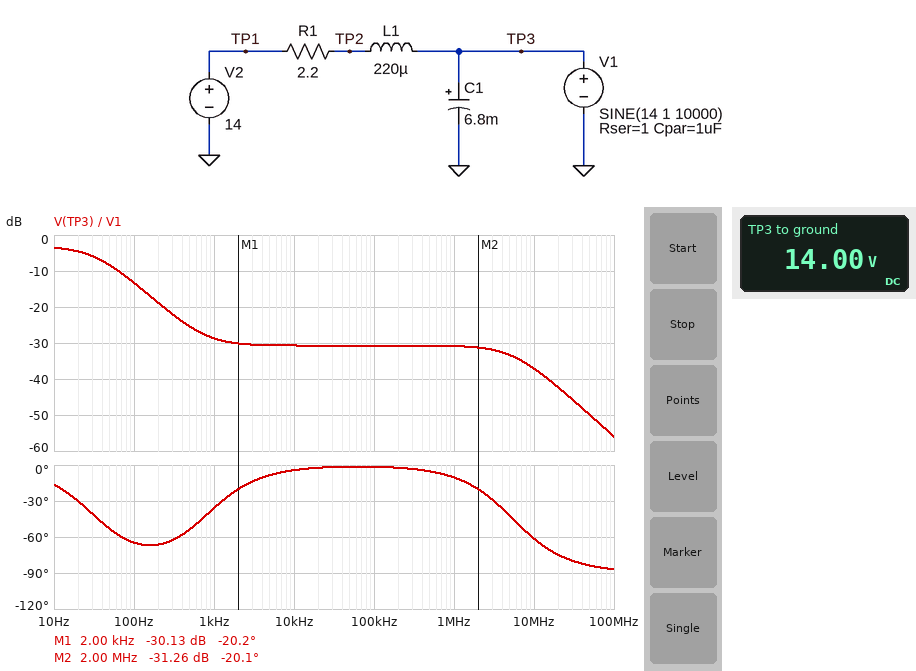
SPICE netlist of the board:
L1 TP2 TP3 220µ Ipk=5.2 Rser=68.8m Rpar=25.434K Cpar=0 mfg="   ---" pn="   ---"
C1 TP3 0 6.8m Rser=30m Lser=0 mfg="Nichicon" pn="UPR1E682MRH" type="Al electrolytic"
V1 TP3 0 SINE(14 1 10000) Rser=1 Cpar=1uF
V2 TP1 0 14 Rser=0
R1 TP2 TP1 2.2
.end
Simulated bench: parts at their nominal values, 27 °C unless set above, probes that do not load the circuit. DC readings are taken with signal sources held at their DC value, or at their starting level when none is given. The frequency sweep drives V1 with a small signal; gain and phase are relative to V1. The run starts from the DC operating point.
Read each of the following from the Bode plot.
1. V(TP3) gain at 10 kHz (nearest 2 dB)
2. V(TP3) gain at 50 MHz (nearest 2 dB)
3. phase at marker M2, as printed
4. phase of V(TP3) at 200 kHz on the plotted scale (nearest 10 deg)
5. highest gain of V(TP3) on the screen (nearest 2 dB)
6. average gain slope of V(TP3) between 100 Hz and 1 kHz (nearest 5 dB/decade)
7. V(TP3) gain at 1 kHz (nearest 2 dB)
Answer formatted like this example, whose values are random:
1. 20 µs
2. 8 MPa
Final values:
1. -30 dB
2. -50 dB
3. -20.1 deg
4. 0 deg
5. -4 dB
6. -15 dB/decade
7. -28 dB
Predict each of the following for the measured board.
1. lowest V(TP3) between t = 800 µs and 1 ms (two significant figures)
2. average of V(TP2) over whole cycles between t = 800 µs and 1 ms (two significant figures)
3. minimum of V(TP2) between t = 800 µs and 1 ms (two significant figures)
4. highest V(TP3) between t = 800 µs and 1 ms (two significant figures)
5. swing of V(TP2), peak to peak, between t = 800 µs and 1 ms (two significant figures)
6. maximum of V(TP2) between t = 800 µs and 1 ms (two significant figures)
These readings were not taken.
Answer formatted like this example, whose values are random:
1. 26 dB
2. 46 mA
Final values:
1. 14 V
2. 14 V
3. 14 V
4. 14 V
5. 9.2 mV
6. 14 V
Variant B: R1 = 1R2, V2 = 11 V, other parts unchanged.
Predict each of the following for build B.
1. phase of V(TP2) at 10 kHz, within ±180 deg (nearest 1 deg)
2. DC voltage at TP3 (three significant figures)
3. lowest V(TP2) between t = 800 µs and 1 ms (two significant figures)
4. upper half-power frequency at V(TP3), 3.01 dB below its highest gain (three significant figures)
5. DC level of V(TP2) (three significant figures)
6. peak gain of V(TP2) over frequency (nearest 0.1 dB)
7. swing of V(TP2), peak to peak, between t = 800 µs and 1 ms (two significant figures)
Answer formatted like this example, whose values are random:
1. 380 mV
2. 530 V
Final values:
1. -89 deg
2. 12.7 V
3. 13 V
4. 40.6 Hz
5. 12.6 V
6. -5.5 dB
7. 5.1 mV
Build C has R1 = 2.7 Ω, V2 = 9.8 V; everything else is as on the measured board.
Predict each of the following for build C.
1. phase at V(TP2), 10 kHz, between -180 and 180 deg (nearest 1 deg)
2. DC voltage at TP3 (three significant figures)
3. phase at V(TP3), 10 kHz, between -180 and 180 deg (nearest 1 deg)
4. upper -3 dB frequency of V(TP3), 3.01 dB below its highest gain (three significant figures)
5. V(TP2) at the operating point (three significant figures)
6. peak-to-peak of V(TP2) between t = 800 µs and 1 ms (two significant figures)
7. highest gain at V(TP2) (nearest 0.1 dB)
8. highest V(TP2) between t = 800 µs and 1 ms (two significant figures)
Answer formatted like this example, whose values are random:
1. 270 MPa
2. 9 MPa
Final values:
1. -83 deg
2. 12.9 V
3. -4 deg
4. 30.8 Hz
5. 12.8 V
6. 11 mV
7. -2.9 dB
8. 13 V
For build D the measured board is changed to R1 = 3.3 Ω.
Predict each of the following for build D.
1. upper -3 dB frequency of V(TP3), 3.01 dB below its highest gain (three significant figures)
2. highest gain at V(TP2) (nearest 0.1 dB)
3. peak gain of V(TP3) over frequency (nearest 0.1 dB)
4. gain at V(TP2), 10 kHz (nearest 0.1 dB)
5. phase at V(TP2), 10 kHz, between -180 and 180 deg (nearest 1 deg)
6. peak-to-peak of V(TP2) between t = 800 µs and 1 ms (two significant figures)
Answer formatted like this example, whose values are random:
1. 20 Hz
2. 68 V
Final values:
1. 29.3 Hz
2. -2.4 dB
3. -2.3 dB
4. -43.4 dB
5. -81 deg
6. 14 mV
